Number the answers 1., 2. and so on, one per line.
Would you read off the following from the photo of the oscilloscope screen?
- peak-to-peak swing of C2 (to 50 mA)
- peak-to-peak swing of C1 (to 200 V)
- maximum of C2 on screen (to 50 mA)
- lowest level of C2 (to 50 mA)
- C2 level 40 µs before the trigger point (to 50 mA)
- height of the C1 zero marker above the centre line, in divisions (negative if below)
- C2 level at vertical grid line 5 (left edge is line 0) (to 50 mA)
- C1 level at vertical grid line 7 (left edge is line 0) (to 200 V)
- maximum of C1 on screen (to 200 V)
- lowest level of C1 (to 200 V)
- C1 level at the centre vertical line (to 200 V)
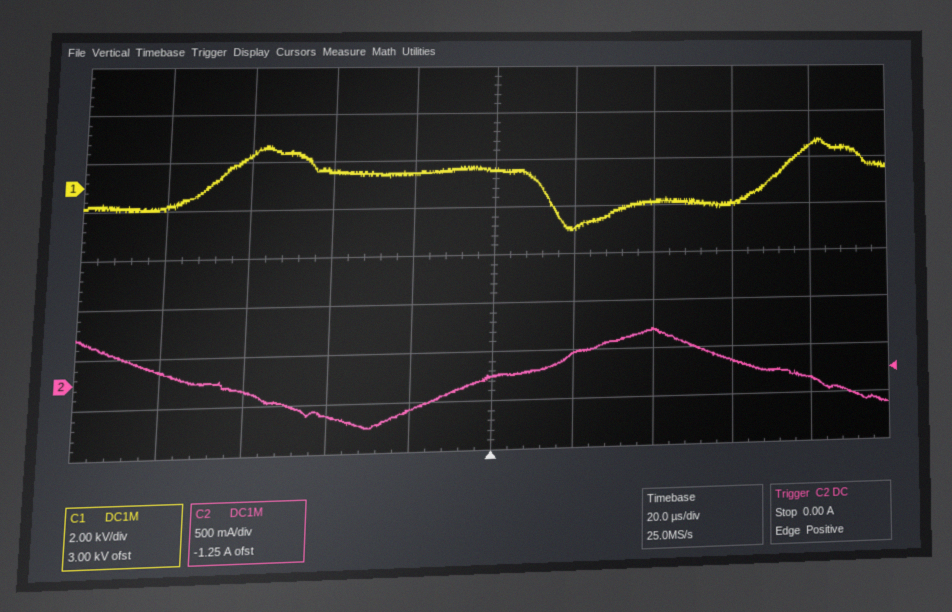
1. 950 mA
2. 3.8 kV
3. 450 mA
4. -500 mA
5. -350 mA
6. +1.5 div
7. 0 mA
8. -800 V
9. 1.8 kV
10. -2.0 kV
11. 600 V
